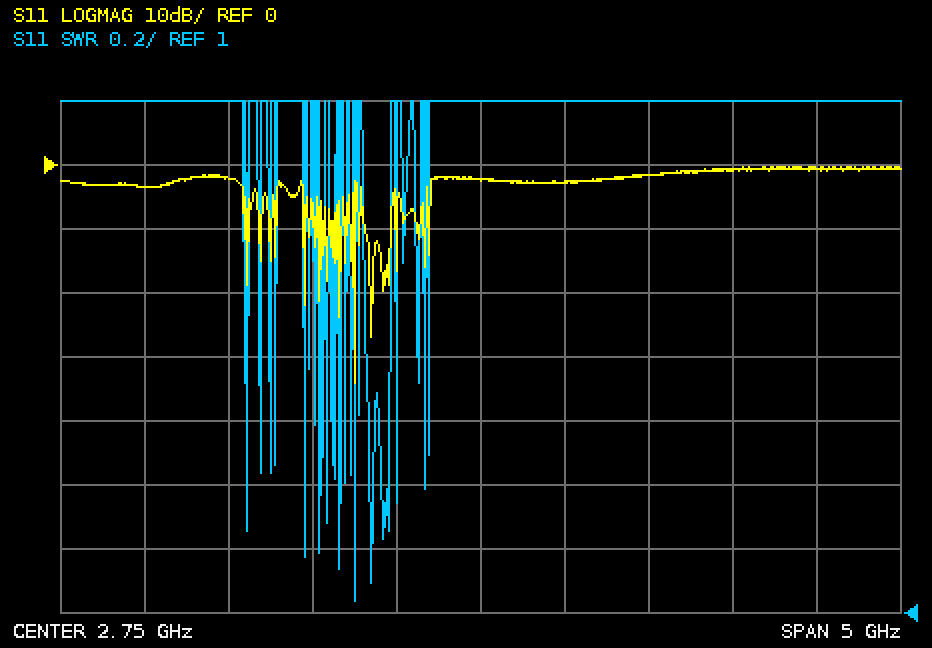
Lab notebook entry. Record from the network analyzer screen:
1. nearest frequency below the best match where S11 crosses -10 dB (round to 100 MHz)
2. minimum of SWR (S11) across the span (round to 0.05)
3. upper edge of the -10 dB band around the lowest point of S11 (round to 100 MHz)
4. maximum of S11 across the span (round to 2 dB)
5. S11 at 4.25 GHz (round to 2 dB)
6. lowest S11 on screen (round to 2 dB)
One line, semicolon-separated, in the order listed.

2.0 GHz; 1.05; 2.0 GHz; 0 dB; 0 dB; -34 dB
